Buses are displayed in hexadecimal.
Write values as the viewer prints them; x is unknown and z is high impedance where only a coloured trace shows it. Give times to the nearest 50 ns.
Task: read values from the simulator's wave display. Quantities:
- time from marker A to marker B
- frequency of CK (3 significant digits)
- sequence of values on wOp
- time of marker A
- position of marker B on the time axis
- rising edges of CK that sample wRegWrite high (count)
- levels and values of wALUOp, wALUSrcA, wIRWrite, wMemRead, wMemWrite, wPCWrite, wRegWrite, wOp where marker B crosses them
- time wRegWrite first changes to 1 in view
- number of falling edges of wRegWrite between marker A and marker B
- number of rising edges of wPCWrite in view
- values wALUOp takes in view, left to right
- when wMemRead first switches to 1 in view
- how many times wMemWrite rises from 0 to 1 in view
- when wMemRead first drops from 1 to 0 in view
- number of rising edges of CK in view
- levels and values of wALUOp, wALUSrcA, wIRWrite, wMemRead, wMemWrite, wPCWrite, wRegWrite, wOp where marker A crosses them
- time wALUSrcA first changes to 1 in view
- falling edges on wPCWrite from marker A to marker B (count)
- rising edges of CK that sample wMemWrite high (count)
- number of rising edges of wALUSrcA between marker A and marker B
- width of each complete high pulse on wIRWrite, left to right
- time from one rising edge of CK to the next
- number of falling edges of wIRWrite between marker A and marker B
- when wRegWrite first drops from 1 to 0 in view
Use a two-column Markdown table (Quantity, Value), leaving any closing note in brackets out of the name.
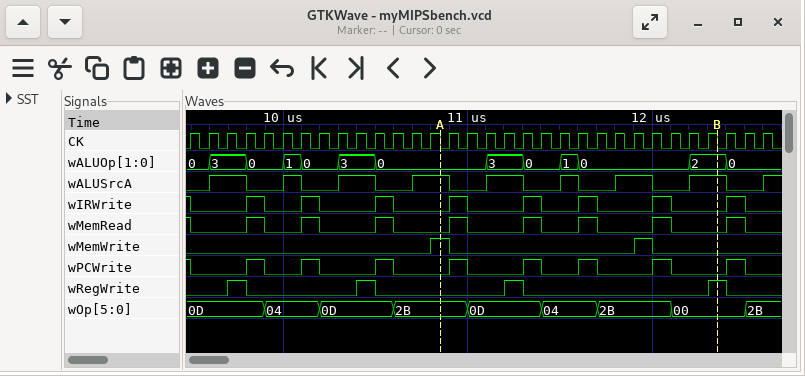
| Quantity | Value |
|---|---|
| time from marker A to marker B | 1500 ns |
| frequency of CK | 10.0 MHz |
| sequence of values on wOp | 0D, 04, 0D, 2B, 0D, 04, 2B, 00, 2B |
| time of marker A | 10850 ns |
| position of marker B on the time axis | 12350 ns |
| rising edges of CK that sample wRegWrite high | 4 |
| levels and values of wALUOp, wALUSrcA, wIRWrite, wMemRead, wMemWrite, wPCWrite, wRegWrite, wOp where marker B crosses them | wALUOp=2, wALUSrcA=1, wIRWrite=0, wMemRead=0, wMemWrite=0, wPCWrite=0, wRegWrite=1, wOp=00 |
| time wRegWrite first changes to 1 in view | 9700 ns |
| number of falling edges of wRegWrite between marker A and marker B | 1 |
| number of rising edges of wPCWrite in view | 8 |
| values wALUOp takes in view, left to right | 0, 3, 0, 1, 0, 3, 0, 3, 0, 1, 0, 2, 0 |
| when wMemRead first switches to 1 in view | 9800 ns |
| how many times wMemWrite rises from 0 to 1 in view | 2 |
| when wMemRead first drops from 1 to 0 in view | 9500 ns |
| number of rising edges of CK in view | 32 |
| levels and values of wALUOp, wALUSrcA, wIRWrite, wMemRead, wMemWrite, wPCWrite, wRegWrite, wOp where marker A crosses them | wALUOp=0, wALUSrcA=1, wIRWrite=0, wMemRead=0, wMemWrite=1, wPCWrite=0, wRegWrite=0, wOp=2B |
| time wALUSrcA first changes to 1 in view | 9600 ns |
| falling edges on wPCWrite from marker A to marker B | 4 |
| rising edges of CK that sample wMemWrite high | 2 |
| number of rising edges of wALUSrcA between marker A and marker B | 4 |
| width of each complete high pulse on wIRWrite, left to right | 100 ns, 100 ns, 100 ns, 100 ns, 100 ns, 100 ns, 100 ns, 100 ns |
| time from one rising edge of CK to the next | 100 ns |
| number of falling edges of wIRWrite between marker A and marker B | 4 |
| when wRegWrite first drops from 1 to 0 in view | 9800 ns |
